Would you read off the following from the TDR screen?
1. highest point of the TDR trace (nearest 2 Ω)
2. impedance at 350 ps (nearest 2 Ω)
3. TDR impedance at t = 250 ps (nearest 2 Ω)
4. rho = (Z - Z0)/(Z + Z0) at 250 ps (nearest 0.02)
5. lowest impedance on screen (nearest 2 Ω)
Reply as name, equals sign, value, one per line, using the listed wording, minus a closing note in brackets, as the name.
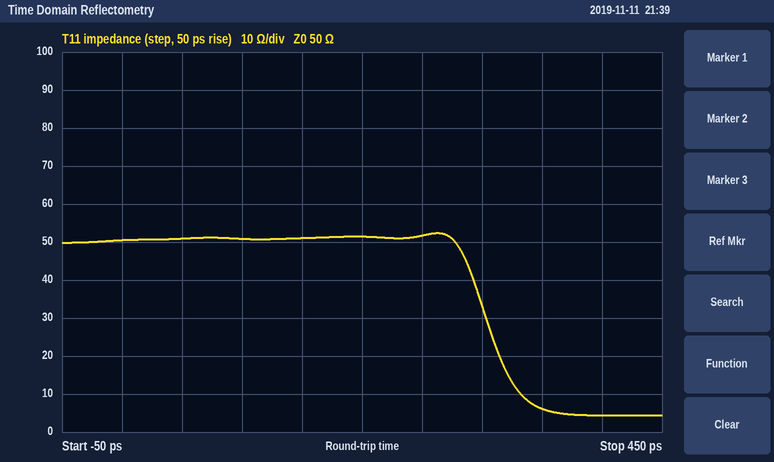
highest point of the TDR trace = 52 Ω
impedance at 350 ps = 6 Ω
TDR impedance at t = 250 ps = 52 Ω
rho = (Z - Z0)/(Z + Z0) at 250 ps = +0.02
lowest impedance on screen = 4 Ω
